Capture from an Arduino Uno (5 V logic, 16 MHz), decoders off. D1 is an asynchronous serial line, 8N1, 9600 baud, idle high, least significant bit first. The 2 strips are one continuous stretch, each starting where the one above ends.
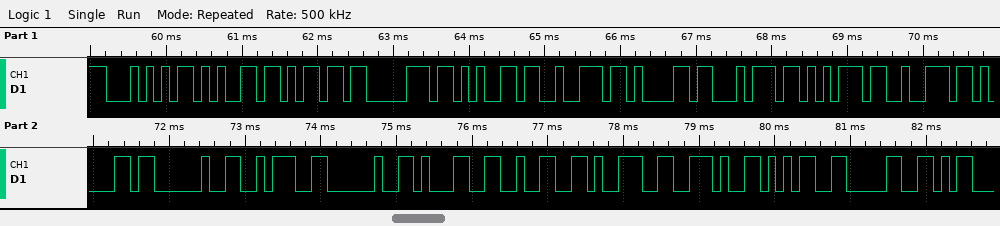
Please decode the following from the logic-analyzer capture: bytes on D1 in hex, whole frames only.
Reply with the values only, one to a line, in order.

54 65 6D 70 65 72 61 74 75 72 61 20 3A 20 31 32 39 2E 35 30
